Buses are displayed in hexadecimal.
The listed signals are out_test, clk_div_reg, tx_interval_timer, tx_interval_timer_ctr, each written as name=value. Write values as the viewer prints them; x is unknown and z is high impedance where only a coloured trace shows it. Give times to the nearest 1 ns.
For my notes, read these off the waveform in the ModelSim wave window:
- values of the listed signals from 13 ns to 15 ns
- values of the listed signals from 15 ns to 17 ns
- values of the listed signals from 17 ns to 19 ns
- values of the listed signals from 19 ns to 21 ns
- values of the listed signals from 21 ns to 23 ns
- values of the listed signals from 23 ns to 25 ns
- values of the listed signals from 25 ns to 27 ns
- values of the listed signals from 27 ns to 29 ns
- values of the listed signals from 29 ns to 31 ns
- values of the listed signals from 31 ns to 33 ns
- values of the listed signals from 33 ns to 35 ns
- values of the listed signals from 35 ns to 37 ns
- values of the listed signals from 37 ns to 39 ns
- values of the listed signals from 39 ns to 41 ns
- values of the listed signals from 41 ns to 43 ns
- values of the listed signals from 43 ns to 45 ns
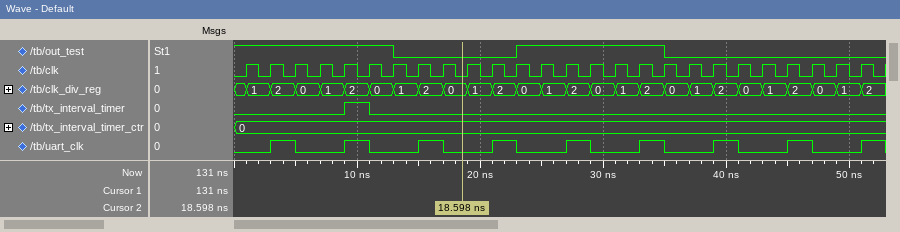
out_test=0, clk_div_reg=1, tx_interval_timer=0, tx_interval_timer_ctr=0
out_test=0, clk_div_reg=2, tx_interval_timer=0, tx_interval_timer_ctr=0
out_test=0, clk_div_reg=0, tx_interval_timer=0, tx_interval_timer_ctr=0
out_test=0, clk_div_reg=1, tx_interval_timer=0, tx_interval_timer_ctr=0
out_test=0, clk_div_reg=2, tx_interval_timer=0, tx_interval_timer_ctr=0
out_test=1, clk_div_reg=0, tx_interval_timer=0, tx_interval_timer_ctr=0
out_test=1, clk_div_reg=1, tx_interval_timer=0, tx_interval_timer_ctr=0
out_test=1, clk_div_reg=2, tx_interval_timer=0, tx_interval_timer_ctr=0
out_test=1, clk_div_reg=0, tx_interval_timer=0, tx_interval_timer_ctr=0
out_test=1, clk_div_reg=1, tx_interval_timer=0, tx_interval_timer_ctr=0
out_test=1, clk_div_reg=2, tx_interval_timer=0, tx_interval_timer_ctr=0
out_test=0, clk_div_reg=0, tx_interval_timer=0, tx_interval_timer_ctr=0
out_test=0, clk_div_reg=1, tx_interval_timer=0, tx_interval_timer_ctr=0
out_test=0, clk_div_reg=2, tx_interval_timer=0, tx_interval_timer_ctr=0
out_test=0, clk_div_reg=0, tx_interval_timer=0, tx_interval_timer_ctr=0
out_test=0, clk_div_reg=1, tx_interval_timer=0, tx_interval_timer_ctr=0
